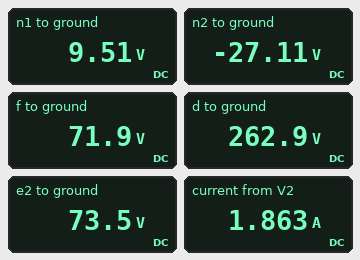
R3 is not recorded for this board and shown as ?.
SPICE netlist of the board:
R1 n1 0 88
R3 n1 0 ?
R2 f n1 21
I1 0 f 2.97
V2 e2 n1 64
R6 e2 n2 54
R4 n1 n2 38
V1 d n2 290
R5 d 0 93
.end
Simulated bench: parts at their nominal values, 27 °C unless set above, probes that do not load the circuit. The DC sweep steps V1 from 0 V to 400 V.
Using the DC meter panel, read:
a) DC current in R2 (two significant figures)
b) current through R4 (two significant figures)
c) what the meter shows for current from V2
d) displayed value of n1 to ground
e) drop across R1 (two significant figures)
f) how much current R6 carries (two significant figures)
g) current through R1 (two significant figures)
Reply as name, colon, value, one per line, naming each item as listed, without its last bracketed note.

DC current in R2: 3.0 A
current through R4: 960 mA
what the meter shows for current from V2: 1.863 A
displayed value of n1 to ground: 9.51 V
drop across R1: 9.5 V
how much current R6 carries: 1.9 A
current through R1: 110 mA
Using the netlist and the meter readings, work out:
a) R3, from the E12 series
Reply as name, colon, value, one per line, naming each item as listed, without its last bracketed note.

R3, from the E12 series: 270 Ω
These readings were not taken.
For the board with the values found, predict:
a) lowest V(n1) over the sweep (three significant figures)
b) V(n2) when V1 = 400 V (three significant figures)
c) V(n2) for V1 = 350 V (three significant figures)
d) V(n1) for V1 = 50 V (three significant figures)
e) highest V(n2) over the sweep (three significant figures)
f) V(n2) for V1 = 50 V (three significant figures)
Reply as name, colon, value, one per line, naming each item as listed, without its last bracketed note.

lowest V(n1) over the sweep: -30.7 V
V(n2) when V1 = 400 V: -80.8 V
V(n2) for V1 = 350 V: -56.4 V
V(n1) for V1 = 50 V: 97.2 V
highest V(n2) over the sweep: 114 V
V(n2) for V1 = 50 V: 90.0 V
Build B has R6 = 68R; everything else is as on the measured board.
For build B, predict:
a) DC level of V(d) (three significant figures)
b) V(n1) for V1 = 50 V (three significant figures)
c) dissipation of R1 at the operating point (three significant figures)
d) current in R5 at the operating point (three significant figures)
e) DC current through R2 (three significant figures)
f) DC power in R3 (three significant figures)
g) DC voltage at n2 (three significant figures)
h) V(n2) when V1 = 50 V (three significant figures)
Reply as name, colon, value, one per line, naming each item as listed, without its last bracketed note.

DC level of V(d): 258 V
V(n1) for V1 = 50 V: 99.6 V
dissipation of R1 at the operating point: 1.89 W
current in R5 at the operating point: 2.78 A
DC current through R2: 2.97 A
DC power in R3: 615 mW
DC voltage at n2: -31.8 V
V(n2) when V1 = 50 V: 86.7 V
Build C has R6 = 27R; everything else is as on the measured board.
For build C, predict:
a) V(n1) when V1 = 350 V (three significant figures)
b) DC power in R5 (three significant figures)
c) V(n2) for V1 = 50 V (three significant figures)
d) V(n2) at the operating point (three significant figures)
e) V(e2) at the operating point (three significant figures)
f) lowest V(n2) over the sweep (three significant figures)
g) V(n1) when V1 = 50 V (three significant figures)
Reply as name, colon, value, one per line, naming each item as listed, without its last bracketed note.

V(n1) when V1 = 350 V: -24.4 V
DC power in R5: 834 W
V(n2) for V1 = 50 V: 101 V
V(n2) at the operating point: -11.5 V
V(e2) at the operating point: 62.4 V
lowest V(n2) over the sweep: -63.1 V
V(n1) when V1 = 50 V: 89.3 V
